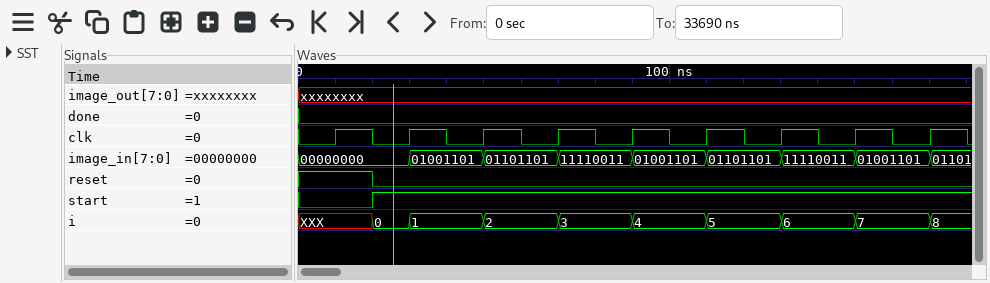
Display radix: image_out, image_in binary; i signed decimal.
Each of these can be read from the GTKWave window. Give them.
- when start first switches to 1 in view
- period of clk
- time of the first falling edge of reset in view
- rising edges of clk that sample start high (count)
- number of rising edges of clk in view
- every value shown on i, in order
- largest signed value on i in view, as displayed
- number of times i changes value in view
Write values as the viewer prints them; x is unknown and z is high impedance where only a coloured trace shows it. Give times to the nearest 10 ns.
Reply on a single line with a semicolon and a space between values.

20 ns; 20 ns; 20 ns; 8; 9; XXX, 0, 1, 2, 3, 4, 5, 6, 7, 8; 8; 9
